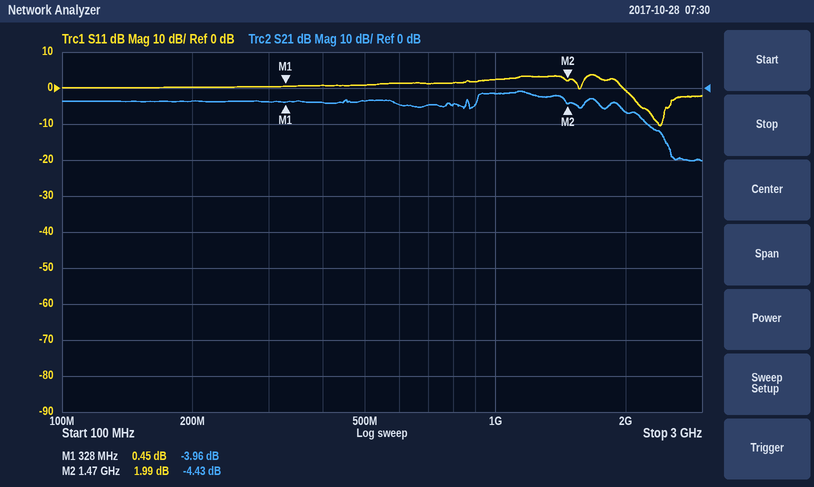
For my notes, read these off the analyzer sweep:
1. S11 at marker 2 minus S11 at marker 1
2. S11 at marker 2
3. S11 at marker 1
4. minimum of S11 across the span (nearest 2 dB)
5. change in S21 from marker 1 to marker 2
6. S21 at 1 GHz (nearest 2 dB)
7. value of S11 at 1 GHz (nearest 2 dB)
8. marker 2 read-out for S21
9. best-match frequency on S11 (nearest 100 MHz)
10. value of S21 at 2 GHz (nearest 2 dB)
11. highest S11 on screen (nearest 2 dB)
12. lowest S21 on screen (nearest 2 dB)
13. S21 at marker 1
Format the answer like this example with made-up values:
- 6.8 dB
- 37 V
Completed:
- 1.54 dB
- 1.99 dB
- 0.45 dB
- -10 dB
- -0.47 dB
- -2 dB
- 2 dB
- -4.43 dB
- 2.4 GHz
- -6 dB
- 4 dB
- -20 dB
- -3.96 dB
